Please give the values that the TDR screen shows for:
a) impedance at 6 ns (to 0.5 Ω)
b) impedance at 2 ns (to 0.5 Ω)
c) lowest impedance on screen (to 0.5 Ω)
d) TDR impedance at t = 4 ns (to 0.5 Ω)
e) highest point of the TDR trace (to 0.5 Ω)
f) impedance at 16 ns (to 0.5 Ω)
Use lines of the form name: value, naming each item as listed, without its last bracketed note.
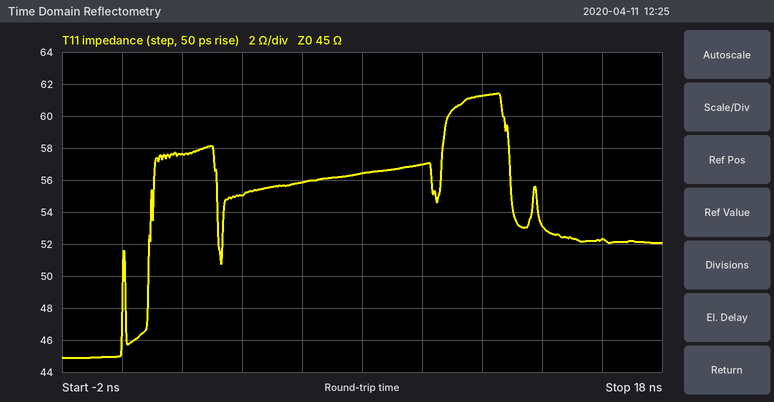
impedance at 6 ns: 56.0 Ω
impedance at 2 ns: 57.5 Ω
lowest impedance on screen: 45.0 Ω
TDR impedance at t = 4 ns: 55.0 Ω
highest point of the TDR trace: 61.5 Ω
impedance at 16 ns: 52.5 Ω
